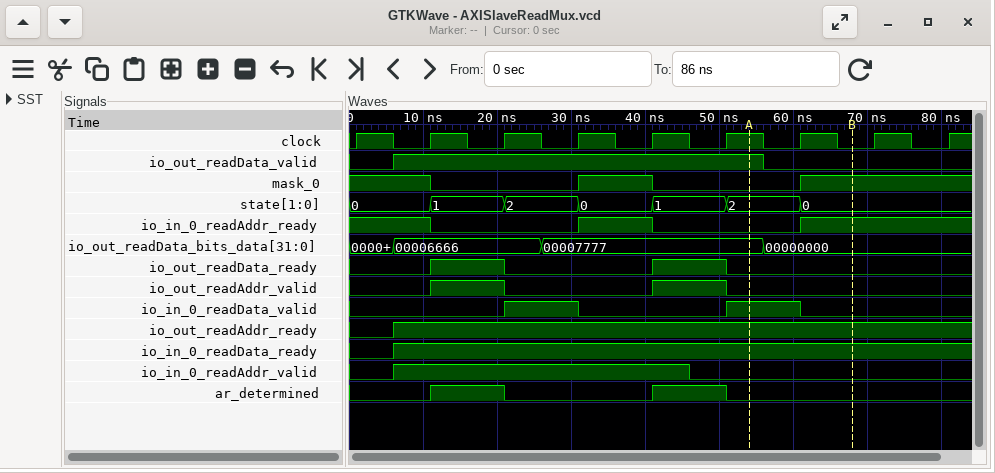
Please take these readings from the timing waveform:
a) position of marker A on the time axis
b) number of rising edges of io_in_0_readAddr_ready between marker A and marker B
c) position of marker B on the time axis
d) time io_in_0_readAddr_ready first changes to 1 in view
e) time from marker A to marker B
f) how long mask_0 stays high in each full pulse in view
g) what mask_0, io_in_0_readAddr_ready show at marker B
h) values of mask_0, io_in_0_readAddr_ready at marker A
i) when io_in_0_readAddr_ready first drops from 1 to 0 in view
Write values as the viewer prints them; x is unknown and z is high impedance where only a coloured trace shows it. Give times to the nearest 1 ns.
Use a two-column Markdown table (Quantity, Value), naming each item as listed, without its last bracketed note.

| Quantity | Value |
|---|---|
| position of marker A on the time axis | 54 ns |
| number of rising edges of io_in_0_readAddr_ready between marker A and marker B | 1 |
| position of marker B on the time axis | 68 ns |
| time io_in_0_readAddr_ready first changes to 1 in view | 31 ns |
| time from marker A to marker B | 14 ns |
| how long mask_0 stays high in each full pulse in view | 10 ns |
| what mask_0, io_in_0_readAddr_ready show at marker B | mask_0=1, io_in_0_readAddr_ready=1 |
| values of mask_0, io_in_0_readAddr_ready at marker A | mask_0=0, io_in_0_readAddr_ready=0 |
| when io_in_0_readAddr_ready first drops from 1 to 0 in view | 11 ns |
